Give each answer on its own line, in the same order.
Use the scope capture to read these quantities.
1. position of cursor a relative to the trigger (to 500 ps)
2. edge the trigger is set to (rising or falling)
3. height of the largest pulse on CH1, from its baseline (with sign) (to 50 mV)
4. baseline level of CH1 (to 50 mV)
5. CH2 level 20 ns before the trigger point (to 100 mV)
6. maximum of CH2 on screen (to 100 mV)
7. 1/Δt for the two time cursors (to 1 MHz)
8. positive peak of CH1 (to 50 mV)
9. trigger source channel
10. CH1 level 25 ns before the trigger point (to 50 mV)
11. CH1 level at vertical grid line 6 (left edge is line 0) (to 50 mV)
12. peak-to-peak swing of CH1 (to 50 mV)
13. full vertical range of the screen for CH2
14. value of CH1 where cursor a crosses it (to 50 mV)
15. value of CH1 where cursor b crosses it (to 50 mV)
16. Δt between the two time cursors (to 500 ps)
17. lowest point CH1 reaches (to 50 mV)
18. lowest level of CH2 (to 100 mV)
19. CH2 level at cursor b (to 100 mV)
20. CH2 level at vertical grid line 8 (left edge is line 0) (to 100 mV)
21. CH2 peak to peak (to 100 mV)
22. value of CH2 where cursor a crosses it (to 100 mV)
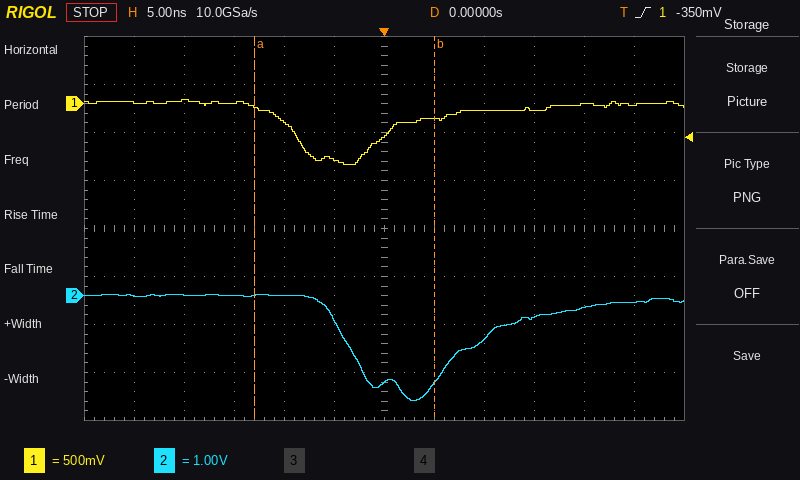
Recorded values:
-13.0 ns
rising
-650 mV
0 mV
0.0 V
0.0 V
56 MHz
50 mV
CH1
0 mV
-350 mV
700 mV
8 V
-50 mV
-150 mV
18.0 ns
-650 mV
-2.2 V
-1.8 V
-900 mV
2.2 V
0.0 V
